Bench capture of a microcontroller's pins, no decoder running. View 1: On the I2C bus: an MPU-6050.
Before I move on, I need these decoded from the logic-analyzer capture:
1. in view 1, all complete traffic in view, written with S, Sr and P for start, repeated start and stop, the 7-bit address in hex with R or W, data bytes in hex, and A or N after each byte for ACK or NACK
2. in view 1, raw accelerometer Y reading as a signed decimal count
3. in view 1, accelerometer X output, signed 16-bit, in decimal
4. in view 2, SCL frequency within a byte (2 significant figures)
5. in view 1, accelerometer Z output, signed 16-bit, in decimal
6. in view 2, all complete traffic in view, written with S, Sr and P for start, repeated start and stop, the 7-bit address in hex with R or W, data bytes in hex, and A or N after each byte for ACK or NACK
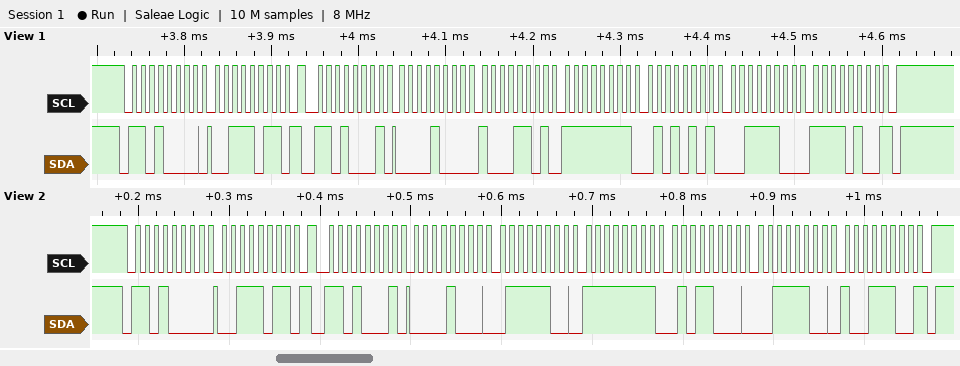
S 68W A 3B A Sr 68R A 08 A 8D A FF A 55 A 3C A F4 N P
-171
2189
100 kHz
15604
S 68W A 3B A Sr 68R A 08 A 7C A FF A 58 A 3C A 9C N P
